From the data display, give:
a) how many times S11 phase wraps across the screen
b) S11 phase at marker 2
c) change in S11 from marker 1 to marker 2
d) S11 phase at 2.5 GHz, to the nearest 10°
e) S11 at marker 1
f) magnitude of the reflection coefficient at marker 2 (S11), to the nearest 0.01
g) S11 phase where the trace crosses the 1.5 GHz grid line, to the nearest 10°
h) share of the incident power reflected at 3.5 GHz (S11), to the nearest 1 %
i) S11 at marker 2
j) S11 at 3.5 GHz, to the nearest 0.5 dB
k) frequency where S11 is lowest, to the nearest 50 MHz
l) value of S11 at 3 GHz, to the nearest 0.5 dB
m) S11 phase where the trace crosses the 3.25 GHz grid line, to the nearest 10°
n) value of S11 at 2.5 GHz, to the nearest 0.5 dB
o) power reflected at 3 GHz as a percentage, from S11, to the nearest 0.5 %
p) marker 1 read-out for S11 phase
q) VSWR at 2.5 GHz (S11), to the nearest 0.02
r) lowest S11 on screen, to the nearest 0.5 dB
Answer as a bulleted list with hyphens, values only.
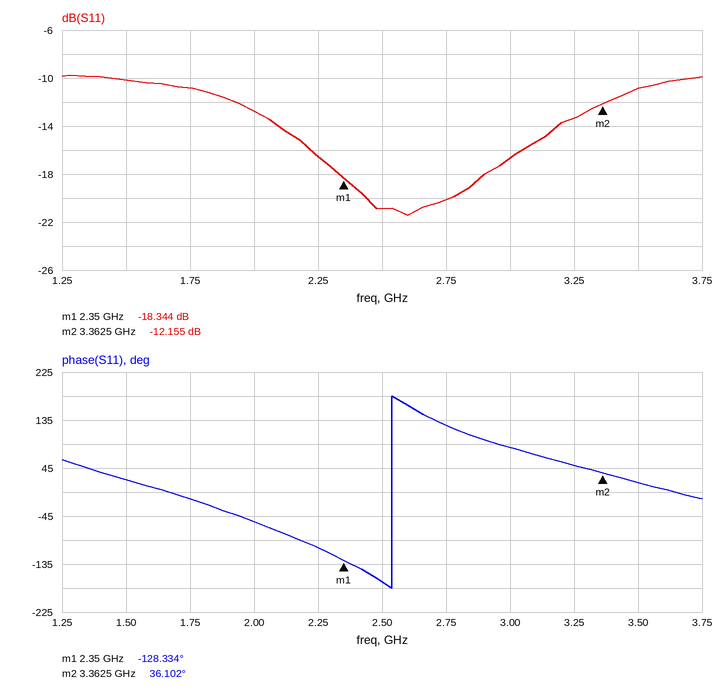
- 1
- 36.102°
- 6.189 dB
- -170°
- -18.344 dB
- 0.25
- 20°
- 8 %
- -12.155 dB
- -11.0 dB
- 2.60 GHz
- -16.5 dB
- 50°
- -21.0 dB
- 2.0 %
- -128.334°
- 1.20
- -21.5 dB
